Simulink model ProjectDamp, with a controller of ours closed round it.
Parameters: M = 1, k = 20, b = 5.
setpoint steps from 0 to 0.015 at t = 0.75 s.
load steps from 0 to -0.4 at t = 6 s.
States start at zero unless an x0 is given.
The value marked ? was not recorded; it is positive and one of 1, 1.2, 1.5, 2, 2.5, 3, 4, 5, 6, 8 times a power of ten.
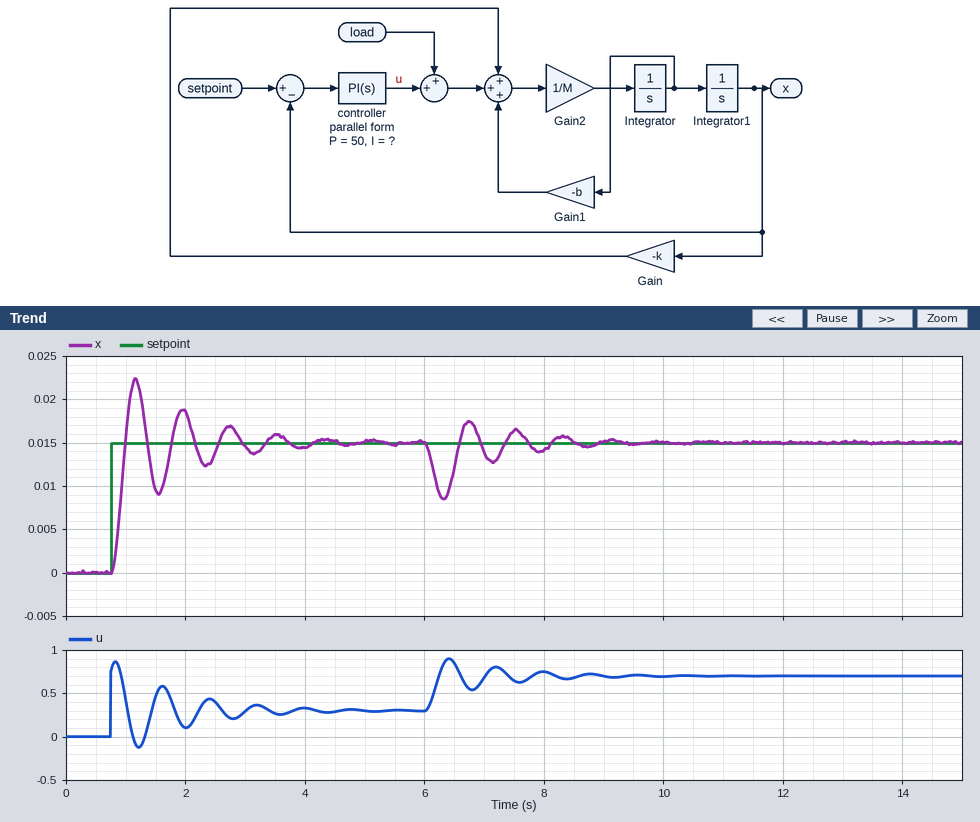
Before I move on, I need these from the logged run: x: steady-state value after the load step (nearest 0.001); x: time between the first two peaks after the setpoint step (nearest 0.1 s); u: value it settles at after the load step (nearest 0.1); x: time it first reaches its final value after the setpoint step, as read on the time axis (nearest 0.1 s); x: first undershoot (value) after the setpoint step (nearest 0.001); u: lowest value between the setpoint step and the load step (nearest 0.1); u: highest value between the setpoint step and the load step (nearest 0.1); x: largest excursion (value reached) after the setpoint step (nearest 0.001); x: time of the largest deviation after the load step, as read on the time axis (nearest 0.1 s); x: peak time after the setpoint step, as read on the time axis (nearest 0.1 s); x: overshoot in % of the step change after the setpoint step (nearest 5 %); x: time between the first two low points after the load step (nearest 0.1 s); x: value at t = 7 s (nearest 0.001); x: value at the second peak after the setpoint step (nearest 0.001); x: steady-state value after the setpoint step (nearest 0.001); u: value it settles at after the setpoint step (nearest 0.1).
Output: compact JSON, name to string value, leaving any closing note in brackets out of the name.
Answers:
{"x: steady-state value after the load step": "0.015", "x: time between the first two peaks after the setpoint step": "0.8 s", "u: value it settles at after the load step": "0.7", "x: time it first reaches its final value after the setpoint step, as read on the time axis": "1.0 s", "x: first undershoot (value) after the setpoint step": "0.009", "u: lowest value between the setpoint step and the load step": "-0.1", "u: highest value between the setpoint step and the load step": "0.9", "x: largest excursion (value reached) after the setpoint step": "0.022", "x: time of the largest deviation after the load step, as read on the time axis": "6.3 s", "x: peak time after the setpoint step, as read on the time axis": "1.2 s", "x: overshoot in % of the step change after the setpoint step": "50 %", "x: time between the first two low points after the load step": "0.8 s", "x: value at t = 7 s": "0.014", "x: value at the second peak after the setpoint step": "0.019", "x: steady-state value after the setpoint step": "0.015", "u: value it settles at after the setpoint step": "0.3"}
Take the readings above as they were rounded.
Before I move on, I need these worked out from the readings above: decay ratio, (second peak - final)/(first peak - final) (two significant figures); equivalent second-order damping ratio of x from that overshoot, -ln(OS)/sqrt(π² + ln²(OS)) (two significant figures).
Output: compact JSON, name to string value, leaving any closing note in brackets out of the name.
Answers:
{"decay ratio, (second peak - final)/(first peak - final)": "0.57", "equivalent second-order damping ratio of x from that overshoot, -ln(OS)/sqrt(π² + ln²(OS))": "0.22"}
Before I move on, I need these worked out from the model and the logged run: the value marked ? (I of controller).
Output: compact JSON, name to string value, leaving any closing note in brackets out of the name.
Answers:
{"the value marked ?": "200"}
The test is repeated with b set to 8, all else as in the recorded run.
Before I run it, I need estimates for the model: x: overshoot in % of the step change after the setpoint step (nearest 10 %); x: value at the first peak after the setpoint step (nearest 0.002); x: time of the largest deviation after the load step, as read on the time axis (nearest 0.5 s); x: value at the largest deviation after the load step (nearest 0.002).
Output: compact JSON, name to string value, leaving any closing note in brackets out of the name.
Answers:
{"x: overshoot in % of the step change after the setpoint step": "30 %", "x: value at the first peak after the setpoint step": "0.020", "x: time of the largest deviation after the load step, as read on the time axis": "6.5 s", "x: value at the largest deviation after the load step": "0.010"}
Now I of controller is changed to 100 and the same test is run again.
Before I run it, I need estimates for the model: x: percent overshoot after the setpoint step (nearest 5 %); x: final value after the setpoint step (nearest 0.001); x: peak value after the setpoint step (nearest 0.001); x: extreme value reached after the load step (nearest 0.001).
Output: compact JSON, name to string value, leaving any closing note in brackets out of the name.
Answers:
{"x: percent overshoot after the setpoint step": "25 %", "x: final value after the setpoint step": "0.015", "x: peak value after the setpoint step": "0.019", "x: extreme value reached after the load step": "0.008"}
